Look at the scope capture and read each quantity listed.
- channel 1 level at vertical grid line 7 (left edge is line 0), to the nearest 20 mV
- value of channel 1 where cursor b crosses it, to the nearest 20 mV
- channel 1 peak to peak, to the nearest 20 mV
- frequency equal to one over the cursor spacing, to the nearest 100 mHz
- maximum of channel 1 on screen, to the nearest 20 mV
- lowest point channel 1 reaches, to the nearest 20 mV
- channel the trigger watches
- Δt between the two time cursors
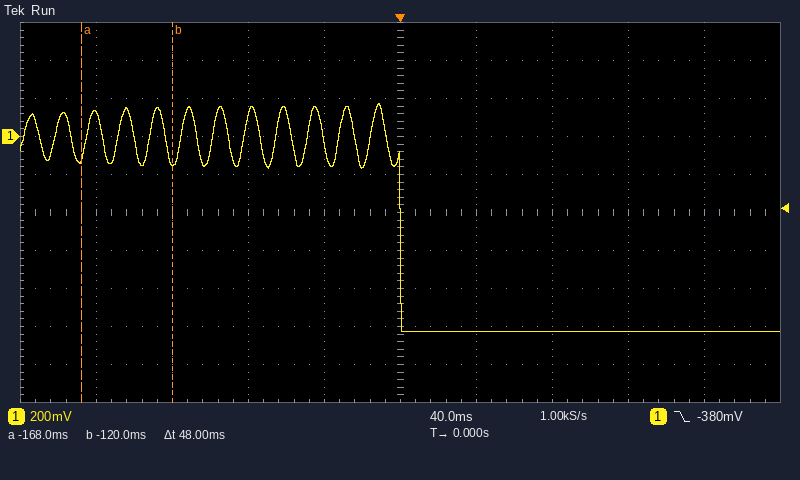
-1.02 V
-140 mV
1.20 V
20.8 Hz
180 mV
-1.02 V
channel 1
48 ms
